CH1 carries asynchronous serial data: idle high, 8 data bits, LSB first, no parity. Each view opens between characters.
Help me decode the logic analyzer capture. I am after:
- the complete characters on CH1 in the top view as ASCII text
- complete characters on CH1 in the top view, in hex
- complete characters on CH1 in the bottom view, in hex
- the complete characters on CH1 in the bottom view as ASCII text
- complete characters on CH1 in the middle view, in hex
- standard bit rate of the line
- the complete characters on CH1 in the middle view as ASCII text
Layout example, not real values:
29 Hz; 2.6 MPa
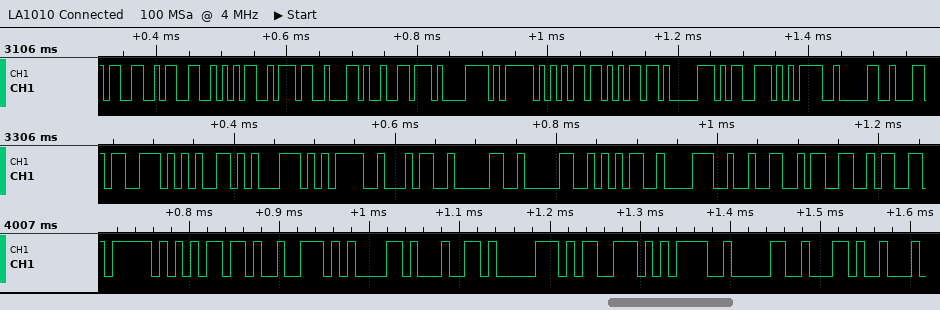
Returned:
"3357,vx_mmps=0"; 33, 33, 35, 37, 2C, 76, 78, 5F, 6D, 6D, 70, 73, 3D, 30; 5F, 6D, 72, 61, 64, 70, 73, 3D, 30, 2C; "_mradps=0,"; 73, 65, 71, 3D, 34, 30, 30, 35, 38, 32, 33; 115200 baud; "seq=4005823"
